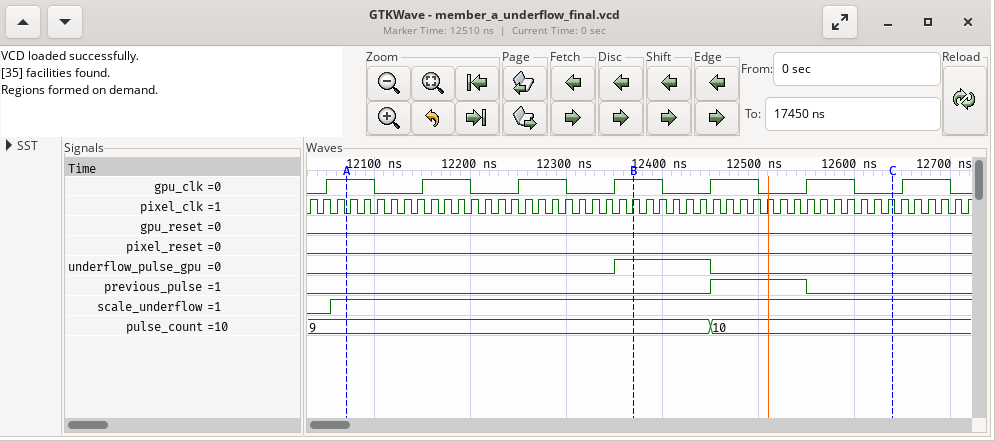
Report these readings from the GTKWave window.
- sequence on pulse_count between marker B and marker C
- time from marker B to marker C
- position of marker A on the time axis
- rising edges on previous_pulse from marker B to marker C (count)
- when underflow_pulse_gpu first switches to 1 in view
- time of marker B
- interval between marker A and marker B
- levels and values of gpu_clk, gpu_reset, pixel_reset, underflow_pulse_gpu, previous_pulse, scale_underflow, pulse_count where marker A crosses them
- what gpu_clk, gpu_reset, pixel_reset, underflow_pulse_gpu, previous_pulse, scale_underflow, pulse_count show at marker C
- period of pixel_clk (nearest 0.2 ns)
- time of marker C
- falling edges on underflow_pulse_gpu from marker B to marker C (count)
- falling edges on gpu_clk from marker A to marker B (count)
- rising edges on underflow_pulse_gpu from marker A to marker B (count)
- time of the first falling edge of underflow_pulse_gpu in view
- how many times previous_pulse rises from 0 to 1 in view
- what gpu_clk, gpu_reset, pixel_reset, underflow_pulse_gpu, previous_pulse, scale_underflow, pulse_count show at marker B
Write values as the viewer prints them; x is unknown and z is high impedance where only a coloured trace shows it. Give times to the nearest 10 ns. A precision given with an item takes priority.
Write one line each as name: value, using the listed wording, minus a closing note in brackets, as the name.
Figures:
sequence on pulse_count between marker B and marker C: 9, 10
time from marker B to marker C: 270 ns
position of marker A on the time axis: 12070 ns
rising edges on previous_pulse from marker B to marker C: 1
when underflow_pulse_gpu first switches to 1 in view: 12350 ns
time of marker B: 12370 ns
interval between marker A and marker B: 300 ns
levels and values of gpu_clk, gpu_reset, pixel_reset, underflow_pulse_gpu, previous_pulse, scale_underflow, pulse_count where marker A crosses them: gpu_clk=1, gpu_reset=0, pixel_reset=0, underflow_pulse_gpu=0, previous_pulse=0, scale_underflow=1, pulse_count=9
what gpu_clk, gpu_reset, pixel_reset, underflow_pulse_gpu, previous_pulse, scale_underflow, pulse_count show at marker C: gpu_clk=0, gpu_reset=0, pixel_reset=0, underflow_pulse_gpu=0, previous_pulse=0, scale_underflow=1, pulse_count=10
period of pixel_clk: 14 ns
time of marker C: 12640 ns
falling edges on underflow_pulse_gpu from marker B to marker C: 1
falling edges on gpu_clk from marker A to marker B: 3
rising edges on underflow_pulse_gpu from marker A to marker B: 1
time of the first falling edge of underflow_pulse_gpu in view: 12450 ns
how many times previous_pulse rises from 0 to 1 in view: 1
what gpu_clk, gpu_reset, pixel_reset, underflow_pulse_gpu, previous_pulse, scale_underflow, pulse_count show at marker B: gpu_clk=1, gpu_reset=0, pixel_reset=0, underflow_pulse_gpu=1, previous_pulse=0, scale_underflow=1, pulse_count=9
